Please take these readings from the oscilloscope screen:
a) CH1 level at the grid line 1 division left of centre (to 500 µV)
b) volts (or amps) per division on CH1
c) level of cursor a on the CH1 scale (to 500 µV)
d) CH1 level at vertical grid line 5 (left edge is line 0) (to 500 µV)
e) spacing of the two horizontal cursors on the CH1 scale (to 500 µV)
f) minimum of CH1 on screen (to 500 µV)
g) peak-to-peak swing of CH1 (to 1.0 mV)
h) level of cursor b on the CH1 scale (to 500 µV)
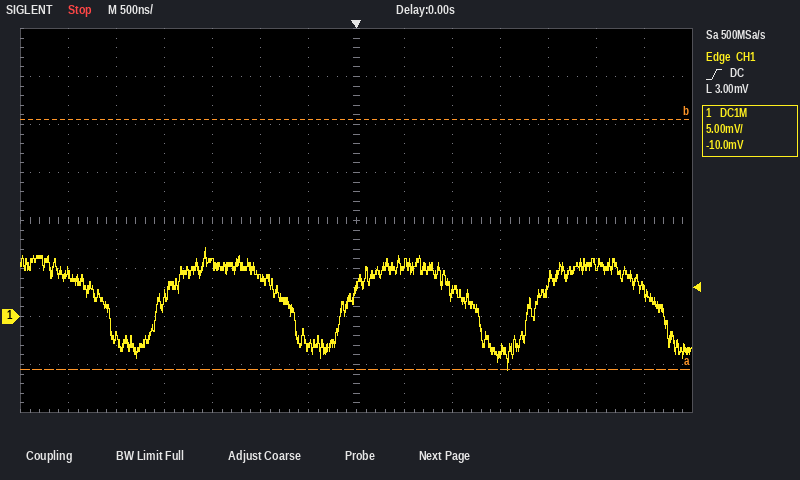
-3.0 mV
5 mV
-5.5 mV
4.0 mV
26.0 mV
-5.5 mV
13.0 mV
20.5 mV
